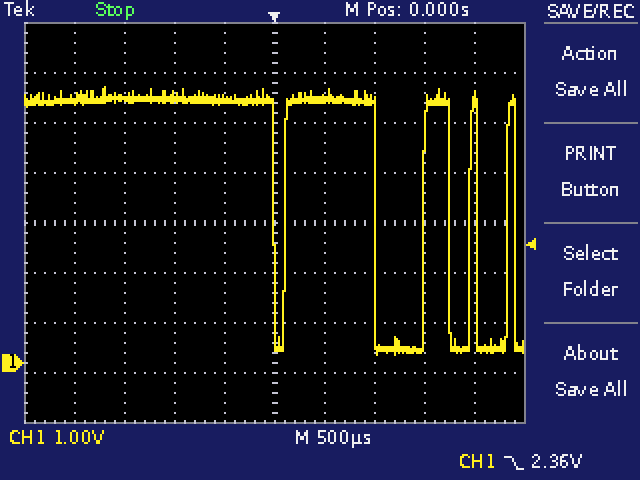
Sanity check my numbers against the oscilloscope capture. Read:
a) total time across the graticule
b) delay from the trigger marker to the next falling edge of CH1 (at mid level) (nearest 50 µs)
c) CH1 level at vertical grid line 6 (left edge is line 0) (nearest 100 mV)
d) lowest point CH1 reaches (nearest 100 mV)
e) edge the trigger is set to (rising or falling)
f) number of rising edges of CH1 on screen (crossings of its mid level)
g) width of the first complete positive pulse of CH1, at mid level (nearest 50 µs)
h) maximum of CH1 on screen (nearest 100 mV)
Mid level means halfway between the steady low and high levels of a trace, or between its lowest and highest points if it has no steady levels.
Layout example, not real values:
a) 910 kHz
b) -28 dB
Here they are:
a) 5 ms
b) 1.00 ms
c) 5.3 V
d) 200 mV
e) falling
f) 4
g) 900 µs
h) 5.5 V
